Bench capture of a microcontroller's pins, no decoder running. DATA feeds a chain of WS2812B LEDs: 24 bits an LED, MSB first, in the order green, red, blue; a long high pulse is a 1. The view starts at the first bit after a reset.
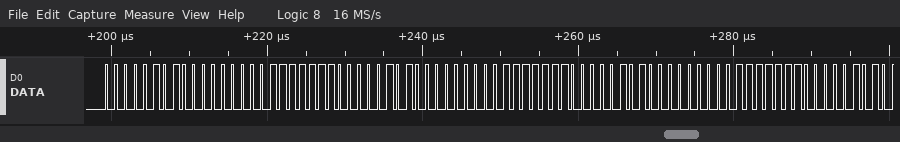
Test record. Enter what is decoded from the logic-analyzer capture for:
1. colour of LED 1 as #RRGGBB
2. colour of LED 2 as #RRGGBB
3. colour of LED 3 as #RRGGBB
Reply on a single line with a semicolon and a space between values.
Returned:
#00057F; #00057F; #00057F
